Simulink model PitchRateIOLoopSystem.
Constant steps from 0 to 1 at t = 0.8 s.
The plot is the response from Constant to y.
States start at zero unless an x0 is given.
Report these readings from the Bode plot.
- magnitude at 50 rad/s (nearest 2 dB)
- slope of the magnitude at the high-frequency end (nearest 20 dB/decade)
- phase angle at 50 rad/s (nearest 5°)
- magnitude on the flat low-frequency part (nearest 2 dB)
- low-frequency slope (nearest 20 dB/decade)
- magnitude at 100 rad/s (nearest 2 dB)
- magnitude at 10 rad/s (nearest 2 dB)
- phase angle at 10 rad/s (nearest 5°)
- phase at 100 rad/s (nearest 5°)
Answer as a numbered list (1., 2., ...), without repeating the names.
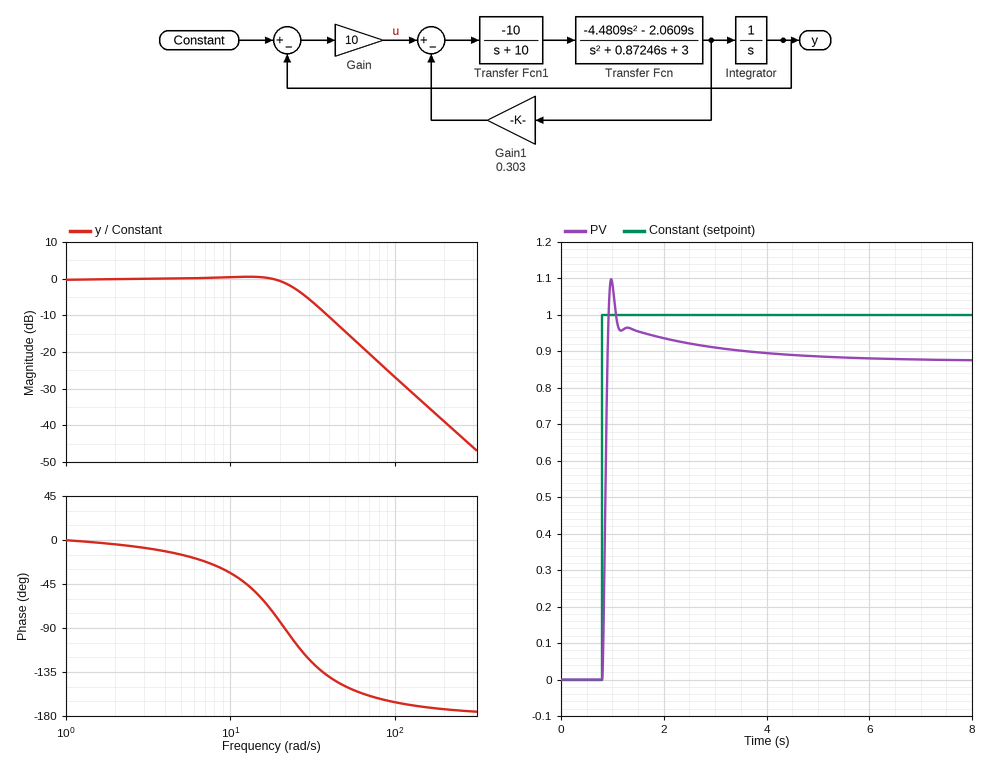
1. -14 dB
2. -40 dB/decade
3. -150°
4. 0 dB
5. 0 dB/decade
6. -26 dB
7. 0 dB
8. -35°
9. -165°
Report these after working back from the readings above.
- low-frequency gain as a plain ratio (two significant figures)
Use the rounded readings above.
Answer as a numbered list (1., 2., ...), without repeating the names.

1. 1.0
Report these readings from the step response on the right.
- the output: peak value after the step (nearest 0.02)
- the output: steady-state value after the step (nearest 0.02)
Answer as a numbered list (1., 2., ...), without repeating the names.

1. 1.10
2. 0.88
